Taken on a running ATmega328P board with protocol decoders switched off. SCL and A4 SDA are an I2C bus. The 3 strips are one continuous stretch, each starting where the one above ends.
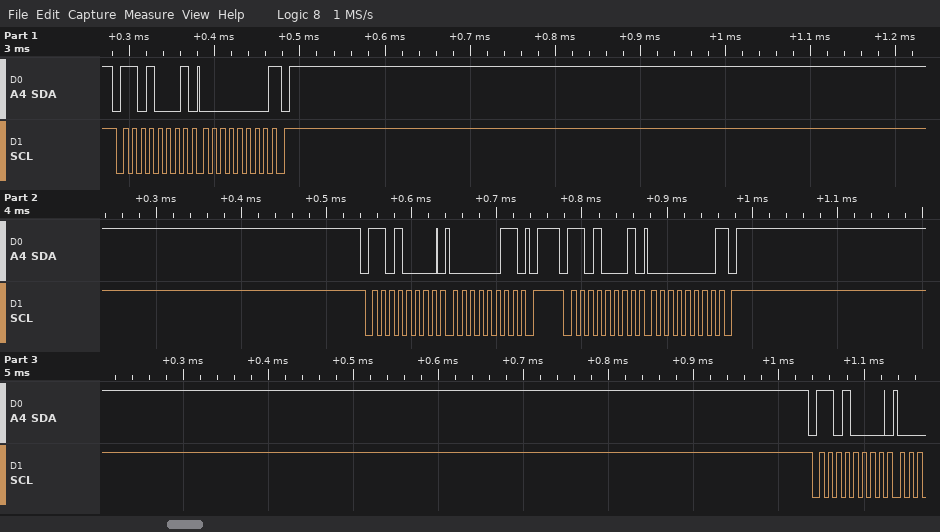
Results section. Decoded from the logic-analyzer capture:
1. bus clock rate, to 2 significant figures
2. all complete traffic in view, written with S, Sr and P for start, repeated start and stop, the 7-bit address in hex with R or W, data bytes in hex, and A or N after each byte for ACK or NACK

100 kHz
S 68R A 00 N P S 68W A 03 A P S 68R A 00 N P S 68W A
